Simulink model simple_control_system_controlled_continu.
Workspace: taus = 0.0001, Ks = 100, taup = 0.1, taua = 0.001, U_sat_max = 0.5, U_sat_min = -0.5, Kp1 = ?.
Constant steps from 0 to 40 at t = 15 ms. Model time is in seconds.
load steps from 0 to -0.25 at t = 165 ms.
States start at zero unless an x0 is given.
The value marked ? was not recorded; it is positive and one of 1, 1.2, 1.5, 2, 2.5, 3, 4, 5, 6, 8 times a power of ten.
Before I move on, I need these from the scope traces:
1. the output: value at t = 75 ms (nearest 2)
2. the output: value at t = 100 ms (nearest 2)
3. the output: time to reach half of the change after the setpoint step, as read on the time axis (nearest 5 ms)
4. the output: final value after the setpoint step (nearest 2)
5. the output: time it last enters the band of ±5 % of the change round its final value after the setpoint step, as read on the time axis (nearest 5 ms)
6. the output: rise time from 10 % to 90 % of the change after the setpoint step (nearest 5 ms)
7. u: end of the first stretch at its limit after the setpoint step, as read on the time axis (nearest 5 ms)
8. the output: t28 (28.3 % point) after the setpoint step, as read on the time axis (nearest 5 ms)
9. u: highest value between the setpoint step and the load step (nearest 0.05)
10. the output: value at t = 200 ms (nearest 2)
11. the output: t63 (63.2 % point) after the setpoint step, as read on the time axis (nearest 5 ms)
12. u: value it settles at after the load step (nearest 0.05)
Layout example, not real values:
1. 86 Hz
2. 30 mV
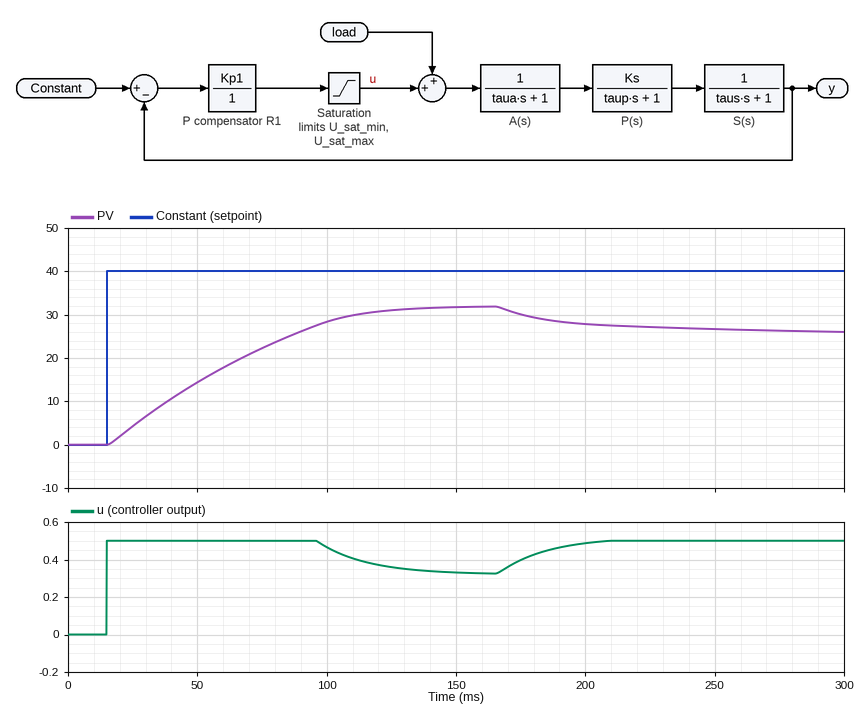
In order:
1. 22
2. 28
3. 55 ms
4. 32
5. 115 ms
6. 80 ms
7. 95 ms
8. 35 ms
9. 0.50
10. 28
11. 70 ms
12. 0.50
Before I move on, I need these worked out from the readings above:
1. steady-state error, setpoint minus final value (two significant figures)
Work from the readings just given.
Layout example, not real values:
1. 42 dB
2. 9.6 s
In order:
1. 8.0
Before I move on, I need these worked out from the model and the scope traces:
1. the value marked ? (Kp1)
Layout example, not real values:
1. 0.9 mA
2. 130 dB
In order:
1. 0.04
